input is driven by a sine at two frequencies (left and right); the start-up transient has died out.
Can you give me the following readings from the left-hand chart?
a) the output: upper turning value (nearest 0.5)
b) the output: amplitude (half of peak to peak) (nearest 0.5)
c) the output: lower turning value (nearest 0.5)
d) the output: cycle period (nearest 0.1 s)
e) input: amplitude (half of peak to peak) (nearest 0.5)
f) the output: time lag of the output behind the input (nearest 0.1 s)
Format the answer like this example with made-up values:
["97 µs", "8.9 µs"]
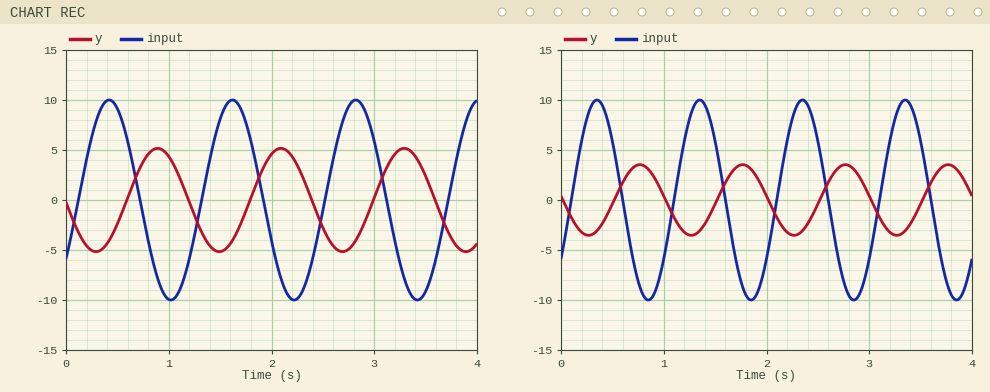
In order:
["5.0", "5.0", "-5.0", "1.2 s", "10.0", "0.5 s"]
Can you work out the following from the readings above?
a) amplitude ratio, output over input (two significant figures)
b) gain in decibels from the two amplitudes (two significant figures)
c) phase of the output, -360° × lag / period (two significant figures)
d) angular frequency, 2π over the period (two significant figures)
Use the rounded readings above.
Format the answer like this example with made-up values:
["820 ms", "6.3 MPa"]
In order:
["0.50", "-6.0 dB", "-150°", "5.2 rad/s"]
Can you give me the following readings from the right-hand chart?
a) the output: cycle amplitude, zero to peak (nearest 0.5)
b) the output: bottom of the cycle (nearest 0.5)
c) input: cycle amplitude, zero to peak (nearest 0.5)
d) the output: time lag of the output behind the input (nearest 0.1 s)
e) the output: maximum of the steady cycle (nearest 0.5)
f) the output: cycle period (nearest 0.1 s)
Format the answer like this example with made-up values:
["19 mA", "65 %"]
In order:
["3.5", "-3.5", "10.0", "0.4 s", "3.5", "1.0 s"]
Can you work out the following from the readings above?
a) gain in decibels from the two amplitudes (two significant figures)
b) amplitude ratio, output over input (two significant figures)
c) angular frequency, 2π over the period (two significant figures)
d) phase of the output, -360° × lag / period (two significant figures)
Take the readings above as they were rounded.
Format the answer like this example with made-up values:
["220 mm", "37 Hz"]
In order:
["-9.1 dB", "0.35", "6.3 rad/s", "-140°"]
